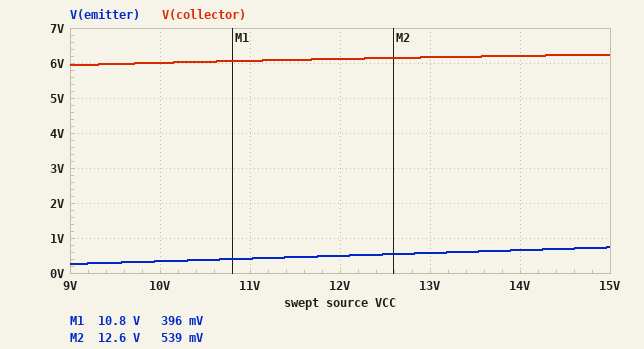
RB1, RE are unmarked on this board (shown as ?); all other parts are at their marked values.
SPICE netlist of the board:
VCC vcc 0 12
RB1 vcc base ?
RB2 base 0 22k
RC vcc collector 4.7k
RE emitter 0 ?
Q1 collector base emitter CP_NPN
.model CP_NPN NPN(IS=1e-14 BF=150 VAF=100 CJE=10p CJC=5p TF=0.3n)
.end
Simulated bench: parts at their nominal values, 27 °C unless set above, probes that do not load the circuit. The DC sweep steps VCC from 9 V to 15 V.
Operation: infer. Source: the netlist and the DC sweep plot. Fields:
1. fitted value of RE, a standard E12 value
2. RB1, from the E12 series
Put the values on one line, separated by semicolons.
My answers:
390 Ω; 180 kΩ
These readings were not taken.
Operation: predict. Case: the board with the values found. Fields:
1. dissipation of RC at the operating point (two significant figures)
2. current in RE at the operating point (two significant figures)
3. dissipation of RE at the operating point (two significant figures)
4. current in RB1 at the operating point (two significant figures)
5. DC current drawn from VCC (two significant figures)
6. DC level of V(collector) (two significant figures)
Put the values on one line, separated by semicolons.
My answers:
7.4 mW; 1.3 mA; 620 µW; 60 µA; 1.3 mA; 6.1 V
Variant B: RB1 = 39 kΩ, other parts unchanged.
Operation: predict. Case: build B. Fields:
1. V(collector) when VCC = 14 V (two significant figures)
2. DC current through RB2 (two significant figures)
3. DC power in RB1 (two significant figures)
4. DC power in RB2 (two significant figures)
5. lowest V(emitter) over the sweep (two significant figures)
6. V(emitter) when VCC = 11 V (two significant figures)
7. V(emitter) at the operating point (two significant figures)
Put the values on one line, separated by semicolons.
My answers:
1.2 V; 76 µA; 2.7 mW; 130 µW; 730 mV; 900 mV; 980 mV
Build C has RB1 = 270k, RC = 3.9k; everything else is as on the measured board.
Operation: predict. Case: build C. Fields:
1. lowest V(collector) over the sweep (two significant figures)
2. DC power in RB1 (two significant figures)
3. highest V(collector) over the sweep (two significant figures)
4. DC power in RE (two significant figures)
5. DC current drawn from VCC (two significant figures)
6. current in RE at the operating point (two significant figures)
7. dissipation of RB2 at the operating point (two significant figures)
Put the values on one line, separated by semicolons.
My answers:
8.4 V; 460 µW; 11 V; 110 µW; 560 µA; 520 µA; 32 µW
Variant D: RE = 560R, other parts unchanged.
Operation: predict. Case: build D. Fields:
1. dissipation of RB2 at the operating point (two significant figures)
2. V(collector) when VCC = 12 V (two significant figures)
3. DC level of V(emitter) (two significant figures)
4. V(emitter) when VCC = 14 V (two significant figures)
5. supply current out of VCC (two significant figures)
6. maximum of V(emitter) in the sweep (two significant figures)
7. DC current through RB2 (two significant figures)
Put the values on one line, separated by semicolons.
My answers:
64 µW; 7.5 V; 540 mV; 710 mV; 1.0 mA; 800 mV; 54 µA
